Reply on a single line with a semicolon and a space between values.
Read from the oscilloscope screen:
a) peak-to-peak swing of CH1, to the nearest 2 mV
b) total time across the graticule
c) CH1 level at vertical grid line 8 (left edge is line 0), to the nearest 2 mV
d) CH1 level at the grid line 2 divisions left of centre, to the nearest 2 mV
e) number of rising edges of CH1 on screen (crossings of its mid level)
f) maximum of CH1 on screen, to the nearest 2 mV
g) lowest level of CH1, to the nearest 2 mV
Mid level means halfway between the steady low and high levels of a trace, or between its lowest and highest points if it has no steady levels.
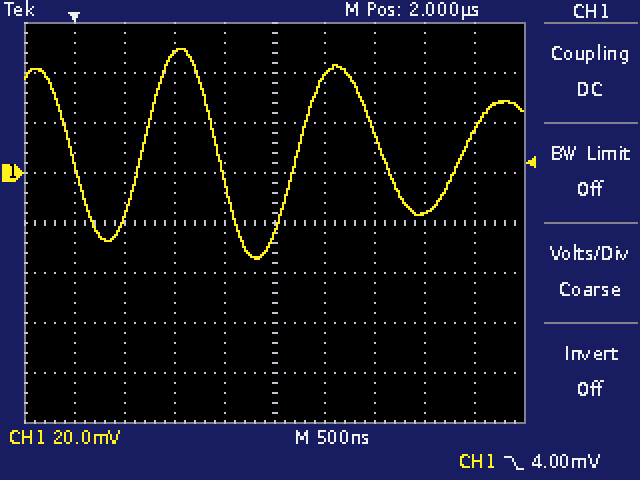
84 mV; 5 µs; -16 mV; 48 mV; 3; 50 mV; -34 mV
